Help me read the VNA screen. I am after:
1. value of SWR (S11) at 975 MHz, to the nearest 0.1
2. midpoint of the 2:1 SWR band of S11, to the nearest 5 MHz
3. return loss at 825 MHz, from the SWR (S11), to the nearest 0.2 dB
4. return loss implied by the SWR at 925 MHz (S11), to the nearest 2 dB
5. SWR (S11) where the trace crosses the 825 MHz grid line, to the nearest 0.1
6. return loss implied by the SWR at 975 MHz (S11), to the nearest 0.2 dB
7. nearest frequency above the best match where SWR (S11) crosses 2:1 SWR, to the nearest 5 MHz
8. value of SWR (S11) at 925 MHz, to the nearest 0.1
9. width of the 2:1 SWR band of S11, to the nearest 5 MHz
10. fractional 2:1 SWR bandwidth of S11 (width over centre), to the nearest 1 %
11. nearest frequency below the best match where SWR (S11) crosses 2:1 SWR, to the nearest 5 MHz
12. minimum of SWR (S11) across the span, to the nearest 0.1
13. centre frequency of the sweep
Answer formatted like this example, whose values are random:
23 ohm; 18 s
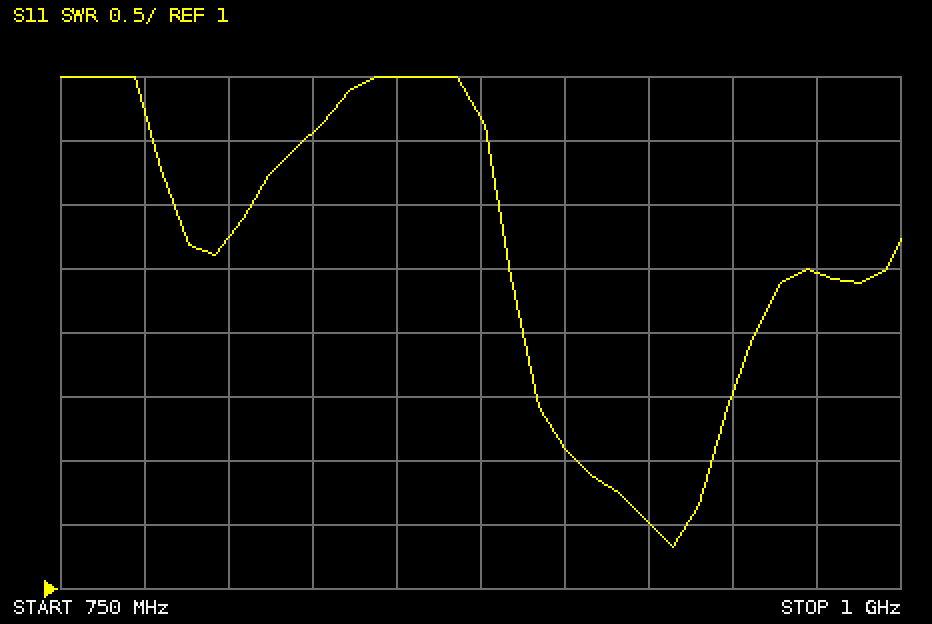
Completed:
3.5; 925 MHz; 3.8 dB; 14 dB; 4.6; 5.2 dB; 945 MHz; 1.5; 40 MHz; 4 %; 905 MHz; 1.3; 875 MHz
